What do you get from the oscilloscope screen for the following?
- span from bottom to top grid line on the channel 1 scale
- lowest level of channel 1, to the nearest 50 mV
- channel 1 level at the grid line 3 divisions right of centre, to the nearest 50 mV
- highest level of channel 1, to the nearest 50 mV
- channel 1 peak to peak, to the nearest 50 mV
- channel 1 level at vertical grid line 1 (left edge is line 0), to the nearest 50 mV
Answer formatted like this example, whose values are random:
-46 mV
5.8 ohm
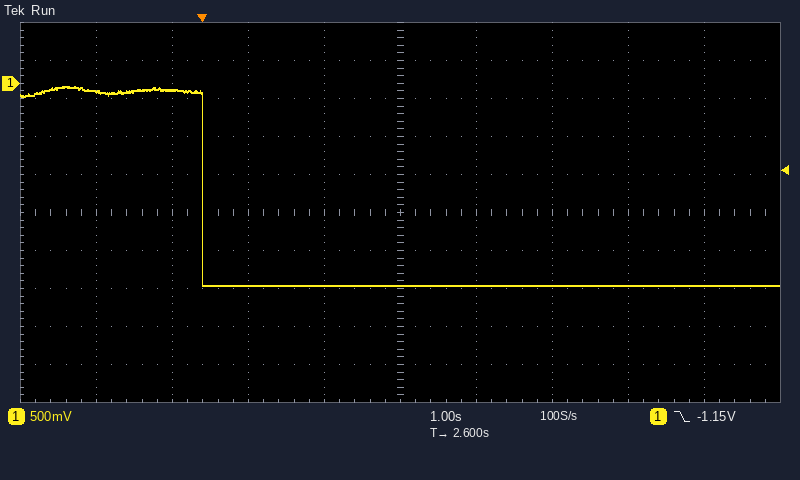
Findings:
5 V
-2.65 V
-2.65 V
-50 mV
2.60 V
-100 mV
